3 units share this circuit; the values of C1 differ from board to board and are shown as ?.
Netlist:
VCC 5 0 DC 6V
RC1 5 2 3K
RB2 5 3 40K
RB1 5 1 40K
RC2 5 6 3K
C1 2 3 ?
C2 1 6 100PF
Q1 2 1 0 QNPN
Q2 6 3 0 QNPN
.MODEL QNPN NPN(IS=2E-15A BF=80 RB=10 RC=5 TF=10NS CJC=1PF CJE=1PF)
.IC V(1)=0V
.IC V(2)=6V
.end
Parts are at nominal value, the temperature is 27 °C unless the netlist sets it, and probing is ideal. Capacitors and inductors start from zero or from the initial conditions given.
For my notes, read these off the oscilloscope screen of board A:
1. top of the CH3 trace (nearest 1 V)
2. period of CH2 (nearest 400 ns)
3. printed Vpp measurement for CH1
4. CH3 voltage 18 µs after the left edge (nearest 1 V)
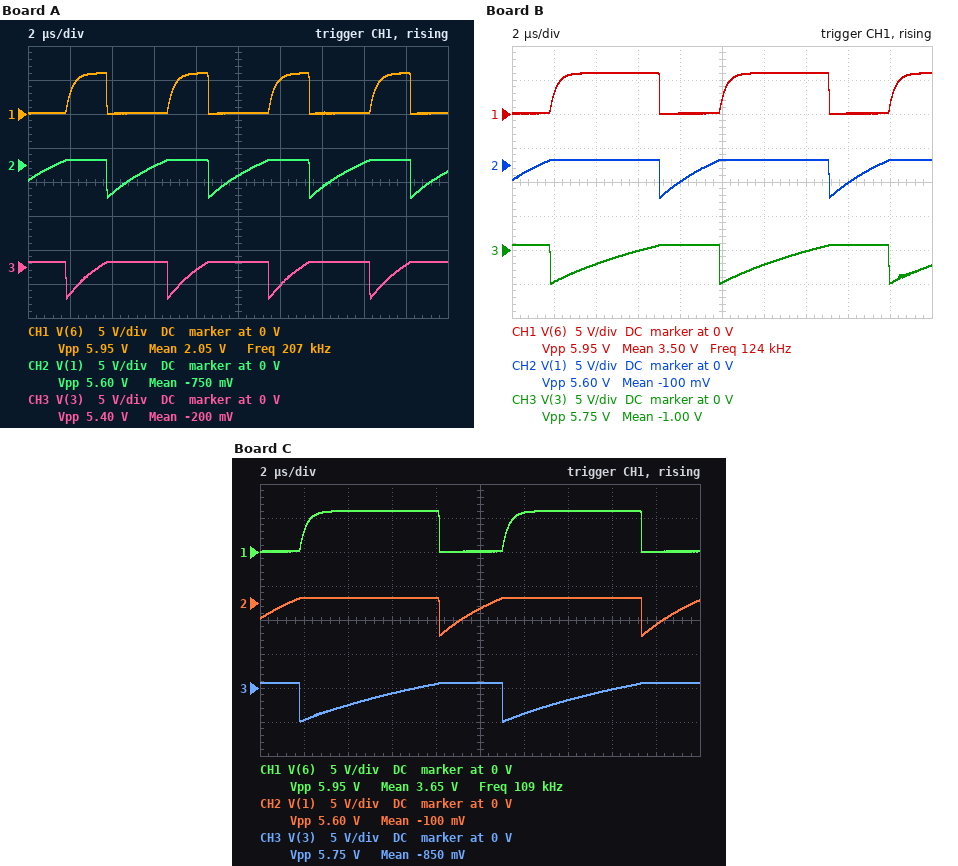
1 V
4.8 µs
5.95 V
0 V
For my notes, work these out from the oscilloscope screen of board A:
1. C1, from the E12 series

68 pF
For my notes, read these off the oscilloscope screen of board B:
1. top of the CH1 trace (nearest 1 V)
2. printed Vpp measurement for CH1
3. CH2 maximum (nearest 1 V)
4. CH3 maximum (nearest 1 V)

6 V
5.95 V
1 V
1 V
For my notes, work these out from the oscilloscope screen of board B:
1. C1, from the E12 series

180 pF
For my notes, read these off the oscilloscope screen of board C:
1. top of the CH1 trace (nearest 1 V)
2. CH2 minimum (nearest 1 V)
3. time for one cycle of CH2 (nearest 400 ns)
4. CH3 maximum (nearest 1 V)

6 V
-5 V
9.2 µs
1 V
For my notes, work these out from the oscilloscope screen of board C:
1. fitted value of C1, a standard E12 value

220 pF
